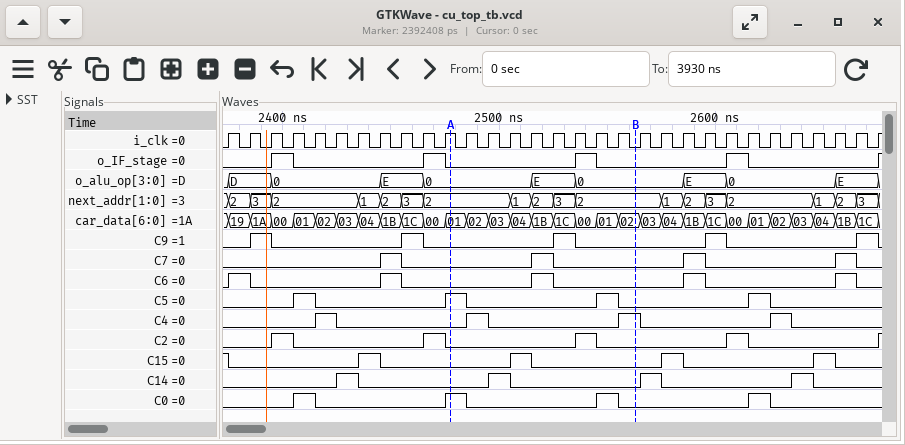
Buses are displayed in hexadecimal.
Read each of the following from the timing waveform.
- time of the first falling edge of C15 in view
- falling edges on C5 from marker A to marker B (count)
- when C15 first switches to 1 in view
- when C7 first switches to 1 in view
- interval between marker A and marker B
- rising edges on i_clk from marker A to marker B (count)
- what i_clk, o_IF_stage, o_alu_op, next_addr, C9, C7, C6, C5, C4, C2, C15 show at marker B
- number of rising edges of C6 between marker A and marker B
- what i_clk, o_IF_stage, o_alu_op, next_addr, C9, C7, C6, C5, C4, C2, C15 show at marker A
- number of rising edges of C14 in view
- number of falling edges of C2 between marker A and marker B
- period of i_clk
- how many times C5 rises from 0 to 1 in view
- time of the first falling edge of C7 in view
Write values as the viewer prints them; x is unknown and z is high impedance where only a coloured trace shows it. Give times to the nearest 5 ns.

2375 ns
2
2435 ns
2445 ns
85 ns
8
i_clk=0, o_IF_stage=0, o_alu_op=0, next_addr=2, C9=0, C7=0, C6=0, C5=0, C4=1, C2=0, C15=0
1
i_clk=1, o_IF_stage=0, o_alu_op=0, next_addr=2, C9=0, C7=0, C6=0, C5=1, C4=0, C2=0, C15=0
4
1
10 ns
4
2455 ns
